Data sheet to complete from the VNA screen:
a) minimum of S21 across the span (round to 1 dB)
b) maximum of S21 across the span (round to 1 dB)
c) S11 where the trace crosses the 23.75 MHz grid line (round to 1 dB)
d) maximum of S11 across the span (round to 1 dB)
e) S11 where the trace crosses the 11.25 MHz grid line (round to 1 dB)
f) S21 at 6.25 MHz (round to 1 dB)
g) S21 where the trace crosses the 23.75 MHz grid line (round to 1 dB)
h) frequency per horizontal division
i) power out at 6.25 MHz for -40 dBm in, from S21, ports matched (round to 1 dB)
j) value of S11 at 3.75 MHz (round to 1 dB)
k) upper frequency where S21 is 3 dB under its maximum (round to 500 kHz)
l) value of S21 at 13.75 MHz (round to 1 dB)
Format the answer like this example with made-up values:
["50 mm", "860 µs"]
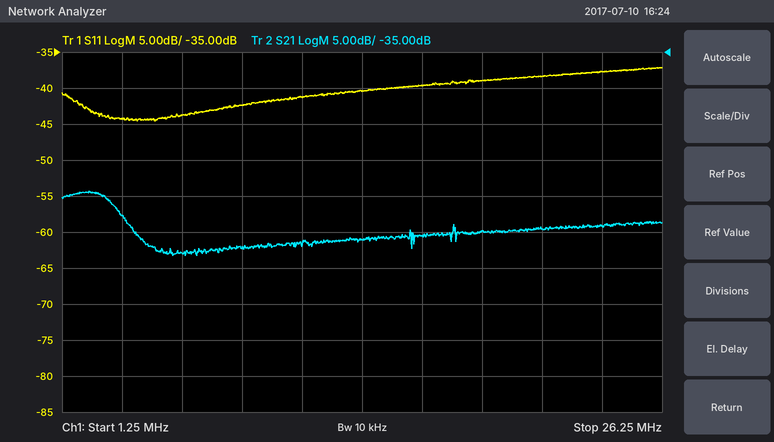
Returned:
["-63 dB", "-54 dB", "-38 dB", "-37 dB", "-41 dB", "-63 dB", "-59 dB", "2.5 MHz", "-103 dBm", "-44 dB", "3.5 MHz", "-61 dB"]
